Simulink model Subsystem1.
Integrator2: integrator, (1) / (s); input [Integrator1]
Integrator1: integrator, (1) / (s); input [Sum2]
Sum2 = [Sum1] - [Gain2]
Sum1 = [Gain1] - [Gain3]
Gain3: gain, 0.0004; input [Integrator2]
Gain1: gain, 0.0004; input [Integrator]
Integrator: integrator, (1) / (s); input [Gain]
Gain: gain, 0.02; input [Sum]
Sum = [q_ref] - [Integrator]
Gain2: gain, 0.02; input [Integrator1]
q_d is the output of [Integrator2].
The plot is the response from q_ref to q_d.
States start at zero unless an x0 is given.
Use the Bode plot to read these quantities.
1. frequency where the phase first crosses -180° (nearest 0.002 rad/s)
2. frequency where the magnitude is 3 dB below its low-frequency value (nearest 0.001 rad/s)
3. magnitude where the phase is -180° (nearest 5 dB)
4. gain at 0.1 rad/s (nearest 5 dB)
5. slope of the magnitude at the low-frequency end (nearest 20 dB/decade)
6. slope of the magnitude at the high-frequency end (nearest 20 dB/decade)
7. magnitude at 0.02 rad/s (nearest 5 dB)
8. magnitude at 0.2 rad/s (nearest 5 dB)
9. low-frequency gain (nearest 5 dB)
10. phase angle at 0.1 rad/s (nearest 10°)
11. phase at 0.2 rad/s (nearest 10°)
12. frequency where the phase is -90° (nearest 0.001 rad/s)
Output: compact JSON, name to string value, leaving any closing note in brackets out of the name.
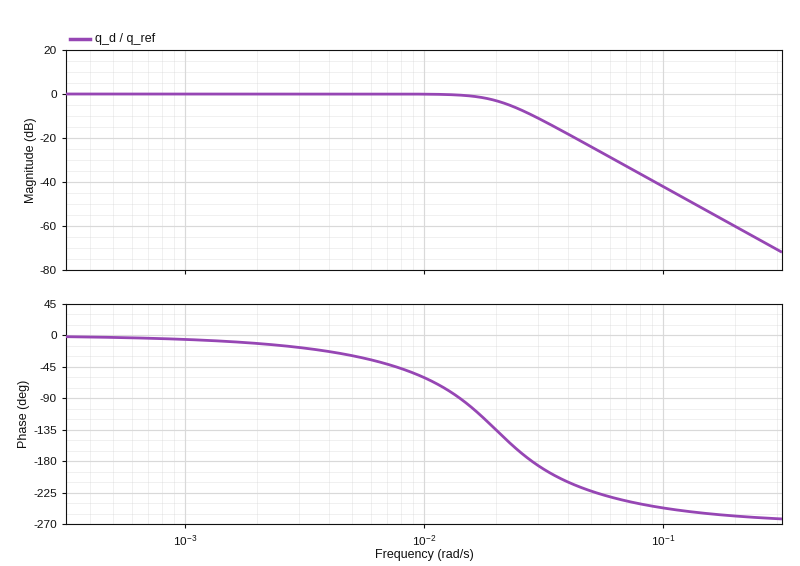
{"frequency where the phase first crosses -180°": "0.028 rad/s", "frequency where the magnitude is 3 dB below its low-frequency value": "0.020 rad/s", "magnitude where the phase is -180°": "-10 dB", "gain at 0.1 rad/s": "-40 dB", "slope of the magnitude at the low-frequency end": "0 dB/decade", "slope of the magnitude at the high-frequency end": "-60 dB/decade", "magnitude at 0.02 rad/s": "-5 dB", "magnitude at 0.2 rad/s": "-60 dB", "low-frequency gain": "0 dB", "phase angle at 0.1 rad/s": "-250°", "phase at 0.2 rad/s": "-260°", "frequency where the phase is -90°": "0.014 rad/s"}
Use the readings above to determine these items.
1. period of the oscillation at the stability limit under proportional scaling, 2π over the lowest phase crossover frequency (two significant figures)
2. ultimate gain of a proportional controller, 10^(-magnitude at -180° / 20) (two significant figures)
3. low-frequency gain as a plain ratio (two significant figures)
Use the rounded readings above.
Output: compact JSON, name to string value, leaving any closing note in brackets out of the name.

{"period of the oscillation at the stability limit under proportional scaling, 2π over the lowest phase crossover frequency": "220 s", "ultimate gain of a proportional controller, 10^(-magnitude at -180° / 20)": "3.2", "low-frequency gain as a plain ratio": "1.0"}
